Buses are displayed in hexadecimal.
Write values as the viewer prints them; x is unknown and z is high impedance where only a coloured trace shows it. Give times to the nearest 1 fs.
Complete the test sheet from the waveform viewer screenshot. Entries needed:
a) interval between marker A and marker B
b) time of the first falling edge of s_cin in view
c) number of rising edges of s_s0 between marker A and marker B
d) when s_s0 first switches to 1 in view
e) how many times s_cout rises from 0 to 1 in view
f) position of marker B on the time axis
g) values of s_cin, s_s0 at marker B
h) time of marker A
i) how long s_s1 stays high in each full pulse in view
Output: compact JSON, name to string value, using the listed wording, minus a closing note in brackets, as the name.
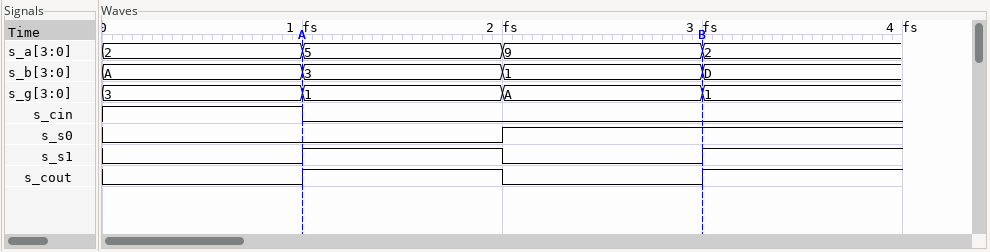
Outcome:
{"interval between marker A and marker B": "2 fs", "time of the first falling edge of s_cin in view": "1 fs", "number of rising edges of s_s0 between marker A and marker B": "1", "when s_s0 first switches to 1 in view": "2 fs", "how many times s_cout rises from 0 to 1 in view": "2", "position of marker B on the time axis": "3 fs", "values of s_cin, s_s0 at marker B": "s_cin=0, s_s0=1", "time of marker A": "1 fs", "how long s_s1 stays high in each full pulse in view": "1 fs"}
